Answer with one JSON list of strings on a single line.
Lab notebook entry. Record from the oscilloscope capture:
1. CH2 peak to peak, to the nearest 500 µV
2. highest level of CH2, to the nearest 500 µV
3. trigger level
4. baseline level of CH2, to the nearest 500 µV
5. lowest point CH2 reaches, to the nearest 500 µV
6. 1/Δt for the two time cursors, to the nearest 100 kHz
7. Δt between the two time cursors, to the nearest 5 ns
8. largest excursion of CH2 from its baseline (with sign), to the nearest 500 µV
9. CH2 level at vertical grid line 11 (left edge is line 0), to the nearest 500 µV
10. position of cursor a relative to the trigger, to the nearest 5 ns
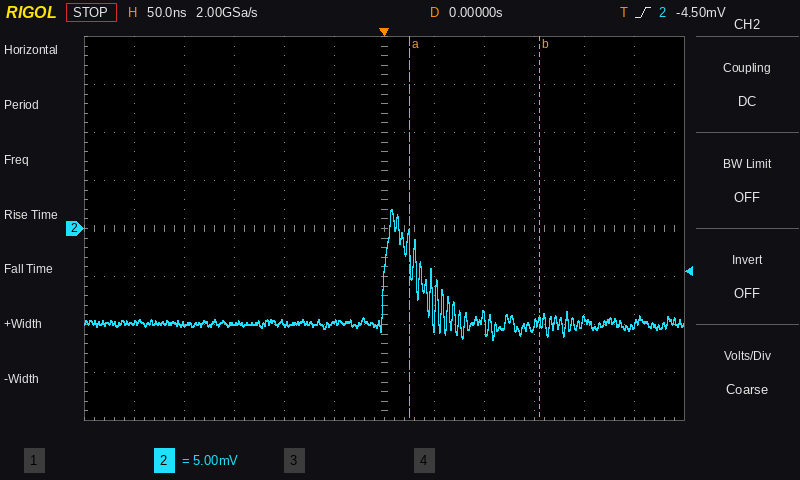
["13.5 mV", "2.0 mV", "-4.50 mV", "-10.0 mV", "-11.5 mV", "7.7 MHz", "130 ns", "+12.0 mV", "-10.0 mV", "+25 ns"]
